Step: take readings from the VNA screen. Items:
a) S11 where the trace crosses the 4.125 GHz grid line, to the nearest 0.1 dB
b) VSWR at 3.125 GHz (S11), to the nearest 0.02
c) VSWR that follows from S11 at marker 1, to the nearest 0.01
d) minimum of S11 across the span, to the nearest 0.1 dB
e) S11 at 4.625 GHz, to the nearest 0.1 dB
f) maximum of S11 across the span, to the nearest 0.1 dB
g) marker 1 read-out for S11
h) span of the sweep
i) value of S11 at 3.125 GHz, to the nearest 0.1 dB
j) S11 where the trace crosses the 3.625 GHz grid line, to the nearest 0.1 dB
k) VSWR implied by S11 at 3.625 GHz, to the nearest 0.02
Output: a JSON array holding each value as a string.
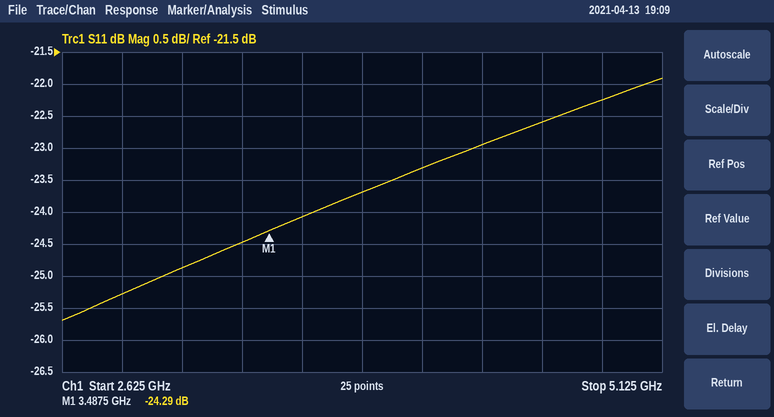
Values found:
["-23.3 dB", "1.12", "1.13", "-25.7 dB", "-22.6 dB", "-21.9 dB", "-24.29 dB", "2.5 GHz", "-24.9 dB", "-24.1 dB", "1.14"]
